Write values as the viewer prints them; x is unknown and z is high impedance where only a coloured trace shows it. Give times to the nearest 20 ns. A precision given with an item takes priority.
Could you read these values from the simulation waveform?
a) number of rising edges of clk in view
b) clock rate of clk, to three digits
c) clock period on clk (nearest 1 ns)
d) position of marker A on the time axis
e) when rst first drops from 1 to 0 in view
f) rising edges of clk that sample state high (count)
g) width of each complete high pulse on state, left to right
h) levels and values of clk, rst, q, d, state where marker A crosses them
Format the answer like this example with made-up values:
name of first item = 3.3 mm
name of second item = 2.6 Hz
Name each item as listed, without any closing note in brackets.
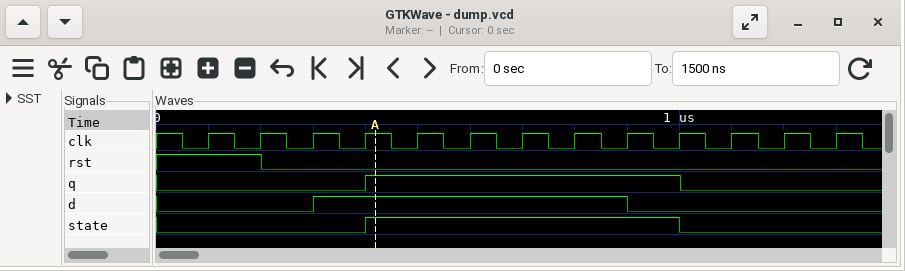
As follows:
number of rising edges of clk in view = 13
clock rate of clk, to three digits = 10.0 MHz
clock period on clk = 100 ns
position of marker A on the time axis = 420 ns
when rst first drops from 1 to 0 in view = 200 ns
rising edges of clk that sample state high = 6
width of each complete high pulse on state, left to right = 600 ns
levels and values of clk, rst, q, d, state where marker A crosses them = clk=1, rst=0, q=1, d=1, state=1
